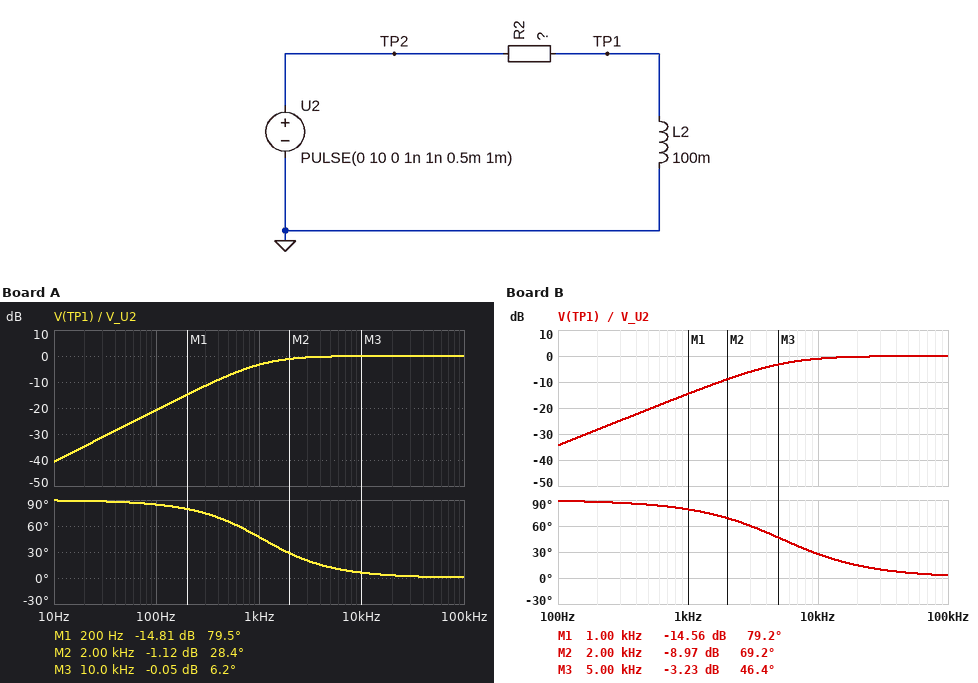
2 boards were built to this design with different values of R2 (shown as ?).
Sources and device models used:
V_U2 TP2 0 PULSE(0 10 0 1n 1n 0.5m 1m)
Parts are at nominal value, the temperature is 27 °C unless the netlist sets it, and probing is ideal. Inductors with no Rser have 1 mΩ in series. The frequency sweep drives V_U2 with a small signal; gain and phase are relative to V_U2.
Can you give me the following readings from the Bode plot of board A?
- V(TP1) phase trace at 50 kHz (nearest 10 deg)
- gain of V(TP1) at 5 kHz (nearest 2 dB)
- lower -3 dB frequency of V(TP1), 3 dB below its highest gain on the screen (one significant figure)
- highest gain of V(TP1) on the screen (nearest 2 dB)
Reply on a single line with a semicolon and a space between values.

0 deg; 0 dB; 1 kHz; 0 dB
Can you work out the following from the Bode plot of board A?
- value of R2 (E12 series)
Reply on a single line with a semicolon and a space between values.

680 Ω
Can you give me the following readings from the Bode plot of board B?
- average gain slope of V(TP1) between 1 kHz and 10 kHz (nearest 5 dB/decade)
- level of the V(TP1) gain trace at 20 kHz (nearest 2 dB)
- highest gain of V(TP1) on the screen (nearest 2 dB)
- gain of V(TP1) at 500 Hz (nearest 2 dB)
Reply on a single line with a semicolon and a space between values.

15 dB/decade; 0 dB; 0 dB; -20 dB
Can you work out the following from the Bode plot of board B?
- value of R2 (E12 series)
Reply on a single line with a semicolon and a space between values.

3.3 kΩ
